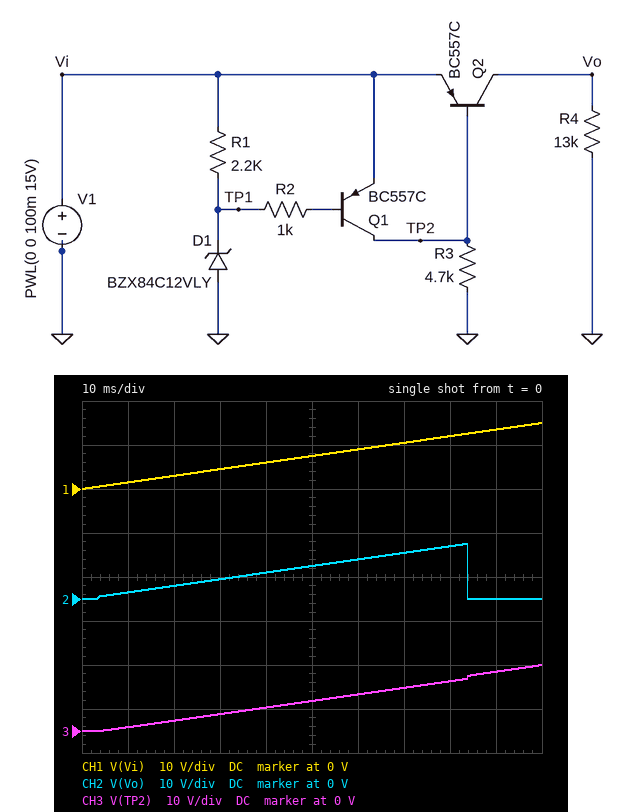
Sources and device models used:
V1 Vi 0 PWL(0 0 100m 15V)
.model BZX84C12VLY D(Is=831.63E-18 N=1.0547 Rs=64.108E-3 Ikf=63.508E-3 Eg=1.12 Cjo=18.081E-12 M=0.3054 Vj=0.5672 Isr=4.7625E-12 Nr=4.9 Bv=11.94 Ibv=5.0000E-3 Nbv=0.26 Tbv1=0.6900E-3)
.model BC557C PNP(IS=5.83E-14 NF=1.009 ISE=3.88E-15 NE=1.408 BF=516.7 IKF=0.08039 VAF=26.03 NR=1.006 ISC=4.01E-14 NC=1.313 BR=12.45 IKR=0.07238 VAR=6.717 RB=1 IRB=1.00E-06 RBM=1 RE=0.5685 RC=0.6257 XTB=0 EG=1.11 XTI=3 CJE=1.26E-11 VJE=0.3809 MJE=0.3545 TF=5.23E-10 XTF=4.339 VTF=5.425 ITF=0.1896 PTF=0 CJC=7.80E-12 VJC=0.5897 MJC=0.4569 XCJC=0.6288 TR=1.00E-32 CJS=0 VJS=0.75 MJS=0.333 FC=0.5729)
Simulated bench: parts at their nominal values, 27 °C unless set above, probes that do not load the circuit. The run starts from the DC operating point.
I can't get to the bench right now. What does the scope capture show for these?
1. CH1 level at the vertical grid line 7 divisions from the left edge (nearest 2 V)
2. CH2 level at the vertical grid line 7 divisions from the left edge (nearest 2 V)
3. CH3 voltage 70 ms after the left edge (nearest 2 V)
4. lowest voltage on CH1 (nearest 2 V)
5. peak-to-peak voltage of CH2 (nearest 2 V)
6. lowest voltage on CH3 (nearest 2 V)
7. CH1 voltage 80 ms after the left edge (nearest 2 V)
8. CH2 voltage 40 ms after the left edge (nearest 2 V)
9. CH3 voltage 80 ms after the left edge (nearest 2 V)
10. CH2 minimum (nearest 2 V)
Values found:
10 V
10 V
10 V
0 V
12 V
0 V
12 V
6 V
12 V
0 V
